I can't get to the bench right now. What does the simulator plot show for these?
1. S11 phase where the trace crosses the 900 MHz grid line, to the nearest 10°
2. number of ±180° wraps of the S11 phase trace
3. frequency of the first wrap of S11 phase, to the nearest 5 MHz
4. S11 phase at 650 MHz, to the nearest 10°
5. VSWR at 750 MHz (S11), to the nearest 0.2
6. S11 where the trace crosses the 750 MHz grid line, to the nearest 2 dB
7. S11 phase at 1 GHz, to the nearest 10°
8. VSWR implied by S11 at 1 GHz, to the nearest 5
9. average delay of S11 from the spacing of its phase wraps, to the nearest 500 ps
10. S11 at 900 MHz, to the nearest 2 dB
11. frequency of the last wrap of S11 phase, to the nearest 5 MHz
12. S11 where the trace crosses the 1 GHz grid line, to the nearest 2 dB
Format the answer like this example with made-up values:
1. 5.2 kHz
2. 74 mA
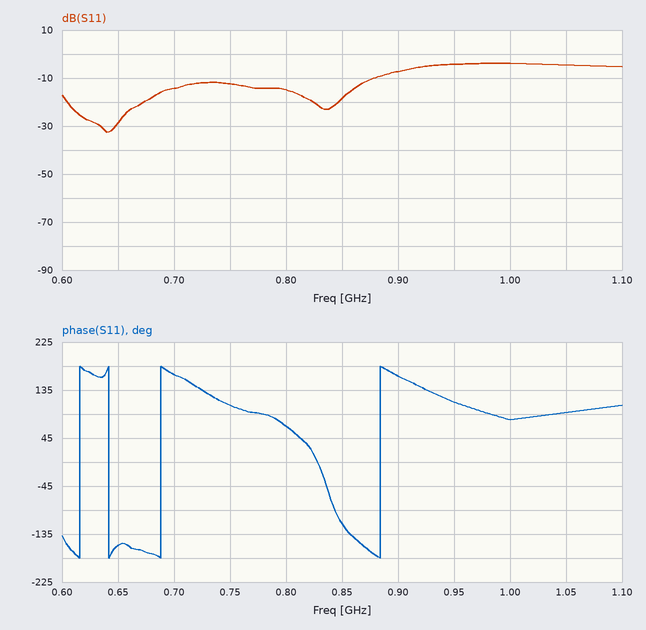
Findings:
1. 160°
2. 4
3. 615 MHz
4. -160°
5. 1.6
6. -12 dB
7. 80°
8. 5
9. 11.0 ns
10. -8 dB
11. 885 MHz
12. -4 dB
